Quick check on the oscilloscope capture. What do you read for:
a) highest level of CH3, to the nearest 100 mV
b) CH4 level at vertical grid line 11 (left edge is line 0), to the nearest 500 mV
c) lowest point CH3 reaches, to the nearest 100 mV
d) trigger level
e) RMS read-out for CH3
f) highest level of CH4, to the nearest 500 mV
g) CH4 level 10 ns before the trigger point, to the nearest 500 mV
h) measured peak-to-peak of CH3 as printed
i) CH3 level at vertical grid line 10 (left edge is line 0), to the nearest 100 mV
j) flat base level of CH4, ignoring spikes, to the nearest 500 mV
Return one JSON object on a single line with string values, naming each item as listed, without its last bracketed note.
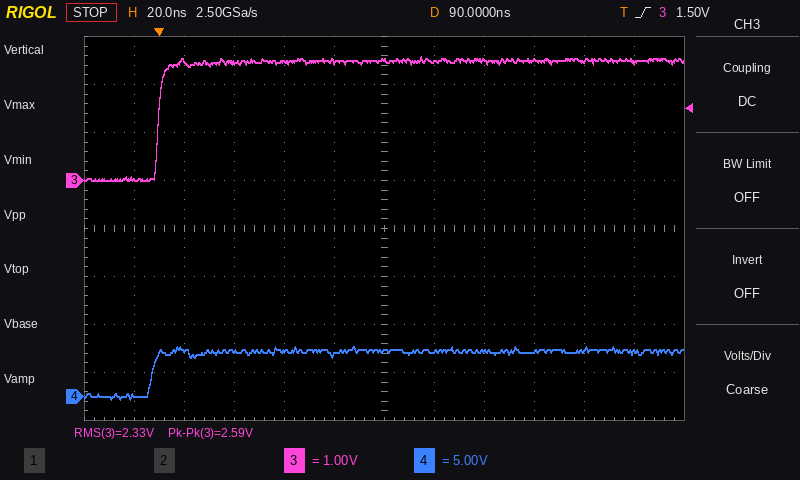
{"highest level of CH3, to the nearest 100 mV": "2.6 V", "CH4 level at vertical grid line 11 (left edge is line 0), to the nearest 500 mV": "4.5 V", "lowest point CH3 reaches, to the nearest 100 mV": "0.0 V", "trigger level": "1.50 V", "RMS read-out for CH3": "2.33 V", "highest level of CH4, to the nearest 500 mV": "5.0 V", "CH4 level 10 ns before the trigger point, to the nearest 500 mV": "0.0 V", "measured peak-to-peak of CH3 as printed": "2.59 V", "CH3 level at vertical grid line 10 (left edge is line 0), to the nearest 100 mV": "2.5 V", "flat base level of CH4, ignoring spikes, to the nearest 500 mV": "0.0 V"}
